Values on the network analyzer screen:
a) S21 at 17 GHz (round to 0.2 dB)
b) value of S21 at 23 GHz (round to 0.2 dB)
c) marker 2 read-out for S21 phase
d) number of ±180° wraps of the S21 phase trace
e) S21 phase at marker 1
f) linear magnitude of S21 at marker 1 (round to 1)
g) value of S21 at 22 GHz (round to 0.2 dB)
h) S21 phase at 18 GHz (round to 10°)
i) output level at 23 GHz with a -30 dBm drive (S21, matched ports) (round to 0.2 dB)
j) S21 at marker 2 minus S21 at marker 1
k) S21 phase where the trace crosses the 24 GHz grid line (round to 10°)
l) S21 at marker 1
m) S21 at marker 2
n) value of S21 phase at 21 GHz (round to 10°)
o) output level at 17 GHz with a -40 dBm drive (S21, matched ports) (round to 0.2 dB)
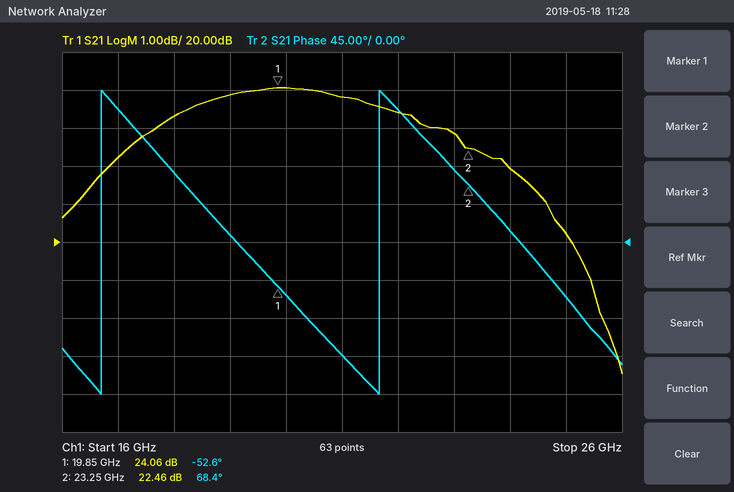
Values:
22.2 dB
22.8 dB
68.4°
2
-52.6°
16
23.4 dB
80°
-7.2 dBm
-1.60 dB
10°
24.06 dB
22.46 dB
-130°
-17.8 dBm
